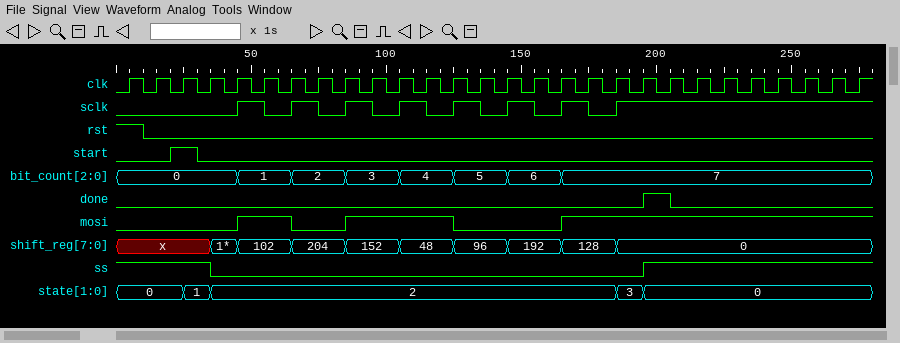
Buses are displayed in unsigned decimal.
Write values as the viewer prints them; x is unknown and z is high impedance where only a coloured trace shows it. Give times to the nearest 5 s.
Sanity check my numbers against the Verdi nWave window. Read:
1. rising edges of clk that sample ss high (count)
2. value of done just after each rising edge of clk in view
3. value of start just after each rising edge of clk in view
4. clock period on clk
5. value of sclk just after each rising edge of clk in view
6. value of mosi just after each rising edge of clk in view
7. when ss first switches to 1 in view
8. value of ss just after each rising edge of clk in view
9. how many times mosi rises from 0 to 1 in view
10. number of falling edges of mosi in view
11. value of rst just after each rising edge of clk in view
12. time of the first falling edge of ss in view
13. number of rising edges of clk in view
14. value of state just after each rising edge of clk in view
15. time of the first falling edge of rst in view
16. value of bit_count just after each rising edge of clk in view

12
0 0 0 0 0 0 0 0 0 0 0 0 0 0 0 0 0 0 0 1 0 0 0 0 0 0 0 0
0 0 1 0 0 0 0 0 0 0 0 0 0 0 0 0 0 0 0 0 0 0 0 0 0 0 0 0
10 s
0 0 0 0 1 0 1 0 1 0 1 0 1 0 1 0 1 0 1 1 1 1 1 1 1 1 1 1
0 0 0 0 1 1 0 0 1 1 1 1 0 0 0 0 1 1 1 1 1 1 1 1 1 1 1 1
195 s
1 1 1 0 0 0 0 0 0 0 0 0 0 0 0 0 0 0 0 1 1 1 1 1 1 1 1 1
3
2
1 0 0 0 0 0 0 0 0 0 0 0 0 0 0 0 0 0 0 0 0 0 0 0 0 0 0 0
35 s
28
0, 0, 1, 2, 2, 2, 2, 2, 2, 2, 2, 2, 2, 2, 2, 2, 2, 2, 3, 0, 0, 0, 0, 0, 0, 0, 0, 0
10 s
0, 0, 0, 0, 1, 1, 2, 2, 3, 3, 4, 4, 5, 5, 6, 6, 7, 7, 7, 7, 7, 7, 7, 7, 7, 7, 7, 7
